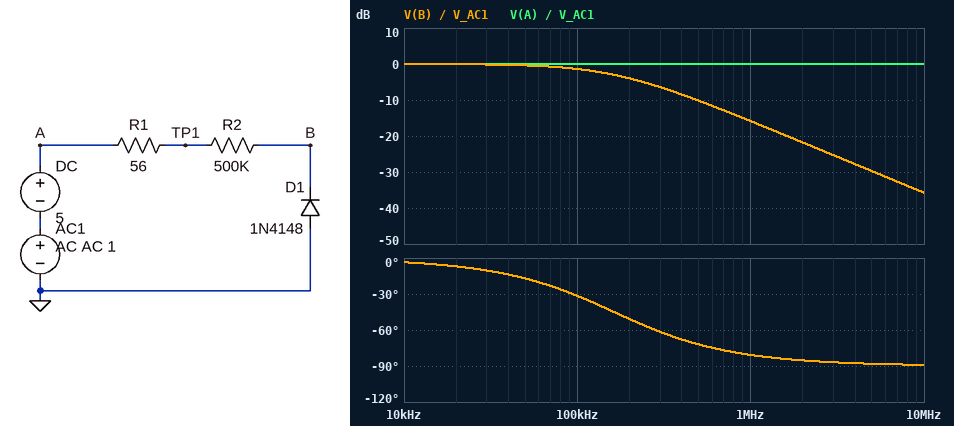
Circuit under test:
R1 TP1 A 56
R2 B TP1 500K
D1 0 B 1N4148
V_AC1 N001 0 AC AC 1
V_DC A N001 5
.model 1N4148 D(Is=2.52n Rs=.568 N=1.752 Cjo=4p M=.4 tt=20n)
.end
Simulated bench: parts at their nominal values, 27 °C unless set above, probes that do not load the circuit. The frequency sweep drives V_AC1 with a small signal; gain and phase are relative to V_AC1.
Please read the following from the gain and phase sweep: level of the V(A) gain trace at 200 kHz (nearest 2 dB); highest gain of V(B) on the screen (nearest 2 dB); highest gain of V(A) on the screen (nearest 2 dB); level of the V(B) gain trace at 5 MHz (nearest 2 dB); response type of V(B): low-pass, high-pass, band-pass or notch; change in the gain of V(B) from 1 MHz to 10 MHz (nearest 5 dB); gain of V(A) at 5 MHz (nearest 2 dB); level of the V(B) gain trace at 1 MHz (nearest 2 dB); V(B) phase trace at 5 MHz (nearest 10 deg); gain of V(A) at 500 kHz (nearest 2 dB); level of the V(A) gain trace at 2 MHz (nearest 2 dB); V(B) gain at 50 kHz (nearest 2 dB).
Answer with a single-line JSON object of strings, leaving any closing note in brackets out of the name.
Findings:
{"level of the V(A) gain trace at 200 kHz": "0 dB", "highest gain of V(B) on the screen": "0 dB", "highest gain of V(A) on the screen": "0 dB", "level of the V(B) gain trace at 5 MHz": "-30 dB", "response type of V(B): low-pass, high-pass, band-pass or notch": "low-pass", "change in the gain of V(B) from 1 MHz to 10 MHz": "-20 dB", "gain of V(A) at 5 MHz": "0 dB", "level of the V(B) gain trace at 1 MHz": "-16 dB", "V(B) phase trace at 5 MHz": "-90 deg", "gain of V(A) at 500 kHz": "0 dB", "level of the V(A) gain trace at 2 MHz": "0 dB", "V(B) gain at 50 kHz": "0 dB"}
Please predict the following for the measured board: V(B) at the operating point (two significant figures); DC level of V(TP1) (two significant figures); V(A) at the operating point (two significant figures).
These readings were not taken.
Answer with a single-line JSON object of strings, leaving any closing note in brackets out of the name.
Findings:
{"V(B) at the operating point": "5.0 V", "DC level of V(TP1)": "5.0 V", "V(A) at the operating point": "5.0 V"}
